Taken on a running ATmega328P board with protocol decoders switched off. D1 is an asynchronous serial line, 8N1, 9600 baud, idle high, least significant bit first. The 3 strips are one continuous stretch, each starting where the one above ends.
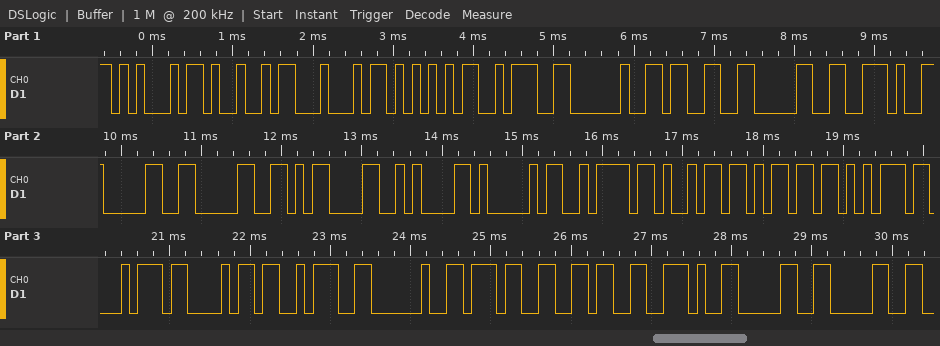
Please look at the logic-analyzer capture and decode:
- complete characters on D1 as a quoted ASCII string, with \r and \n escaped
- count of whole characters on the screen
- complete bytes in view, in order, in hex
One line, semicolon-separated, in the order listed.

"EIDU: 30.00\r\nAzimuth: 76.00"; 27; 45 49 44 55 3A 20 33 30 2E 30 30 0D 0A 41 7A 69 6D 75 74 68 3A 20 37 36 2E 30 30
